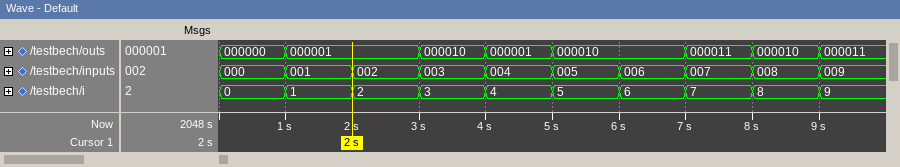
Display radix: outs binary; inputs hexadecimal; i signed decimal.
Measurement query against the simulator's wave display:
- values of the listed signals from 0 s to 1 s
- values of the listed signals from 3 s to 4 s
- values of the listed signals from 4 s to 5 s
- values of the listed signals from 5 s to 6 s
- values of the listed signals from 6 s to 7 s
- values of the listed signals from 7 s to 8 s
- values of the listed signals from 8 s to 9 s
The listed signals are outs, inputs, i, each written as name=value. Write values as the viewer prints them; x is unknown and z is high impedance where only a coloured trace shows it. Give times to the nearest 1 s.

outs=000000, inputs=000, i=0
outs=000010, inputs=003, i=3
outs=000001, inputs=004, i=4
outs=000010, inputs=005, i=5
outs=000010, inputs=006, i=6
outs=000011, inputs=007, i=7
outs=000010, inputs=008, i=8
